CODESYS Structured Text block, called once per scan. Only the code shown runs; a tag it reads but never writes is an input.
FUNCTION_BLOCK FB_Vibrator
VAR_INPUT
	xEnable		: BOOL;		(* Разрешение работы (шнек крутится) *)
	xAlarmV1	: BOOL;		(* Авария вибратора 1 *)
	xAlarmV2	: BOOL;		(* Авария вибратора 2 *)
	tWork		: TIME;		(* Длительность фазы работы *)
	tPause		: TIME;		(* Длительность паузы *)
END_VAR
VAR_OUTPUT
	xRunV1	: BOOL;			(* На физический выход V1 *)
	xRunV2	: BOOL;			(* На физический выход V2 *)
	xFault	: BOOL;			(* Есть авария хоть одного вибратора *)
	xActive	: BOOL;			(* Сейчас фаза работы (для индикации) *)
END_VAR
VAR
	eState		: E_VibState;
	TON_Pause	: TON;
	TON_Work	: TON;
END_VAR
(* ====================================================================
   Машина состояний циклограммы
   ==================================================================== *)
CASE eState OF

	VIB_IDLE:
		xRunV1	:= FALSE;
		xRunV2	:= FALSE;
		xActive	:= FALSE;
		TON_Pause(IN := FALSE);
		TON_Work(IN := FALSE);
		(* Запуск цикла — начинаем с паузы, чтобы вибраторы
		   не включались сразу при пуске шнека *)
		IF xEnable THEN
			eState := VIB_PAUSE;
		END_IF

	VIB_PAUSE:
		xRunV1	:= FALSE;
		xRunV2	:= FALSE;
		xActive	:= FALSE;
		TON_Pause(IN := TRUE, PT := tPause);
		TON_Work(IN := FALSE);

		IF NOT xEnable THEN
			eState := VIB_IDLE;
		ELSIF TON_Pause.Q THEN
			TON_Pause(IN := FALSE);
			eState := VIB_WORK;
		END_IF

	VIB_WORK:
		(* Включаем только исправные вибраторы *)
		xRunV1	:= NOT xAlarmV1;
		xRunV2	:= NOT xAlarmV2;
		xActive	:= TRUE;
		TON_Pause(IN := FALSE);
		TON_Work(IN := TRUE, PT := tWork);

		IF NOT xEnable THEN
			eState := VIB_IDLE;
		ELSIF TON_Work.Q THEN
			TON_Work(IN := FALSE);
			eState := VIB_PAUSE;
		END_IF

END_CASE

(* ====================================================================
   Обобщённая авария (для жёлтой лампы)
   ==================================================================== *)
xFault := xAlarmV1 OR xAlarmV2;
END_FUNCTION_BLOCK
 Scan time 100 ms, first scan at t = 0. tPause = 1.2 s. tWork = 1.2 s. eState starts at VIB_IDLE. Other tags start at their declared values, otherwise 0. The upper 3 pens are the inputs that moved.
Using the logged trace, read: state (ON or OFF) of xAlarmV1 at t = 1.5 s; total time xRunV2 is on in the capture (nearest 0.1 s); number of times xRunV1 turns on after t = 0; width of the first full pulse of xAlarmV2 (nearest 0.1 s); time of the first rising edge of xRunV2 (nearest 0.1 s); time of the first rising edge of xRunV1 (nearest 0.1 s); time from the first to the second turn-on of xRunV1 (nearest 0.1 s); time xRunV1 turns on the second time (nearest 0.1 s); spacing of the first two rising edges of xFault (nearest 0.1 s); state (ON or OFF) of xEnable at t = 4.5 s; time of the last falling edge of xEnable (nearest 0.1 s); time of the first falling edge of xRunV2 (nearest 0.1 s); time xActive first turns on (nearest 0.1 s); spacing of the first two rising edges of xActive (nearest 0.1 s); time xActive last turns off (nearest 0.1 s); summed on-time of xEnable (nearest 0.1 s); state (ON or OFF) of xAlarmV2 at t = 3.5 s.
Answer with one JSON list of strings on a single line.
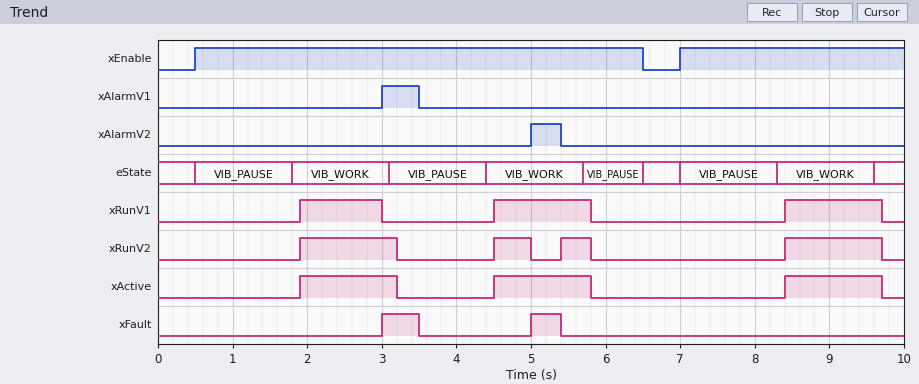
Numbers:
["OFF", "3.5 s", "3", "0.4 s", "1.9 s", "1.9 s", "2.6 s", "4.5 s", "2.0 s", "ON", "6.5 s", "3.2 s", "1.9 s", "2.6 s", "9.7 s", "9.0 s", "OFF"]
